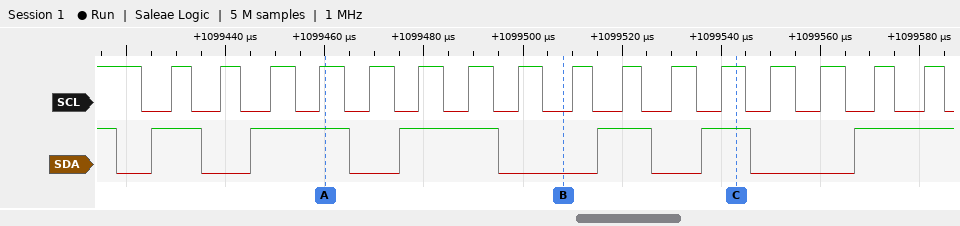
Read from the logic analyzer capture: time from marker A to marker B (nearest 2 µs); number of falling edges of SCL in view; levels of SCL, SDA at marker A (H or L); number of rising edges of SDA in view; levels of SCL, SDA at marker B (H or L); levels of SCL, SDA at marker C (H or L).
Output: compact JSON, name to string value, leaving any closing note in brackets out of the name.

{"time from marker A to marker B": "48 µs", "number of falling edges of SCL in view": "17", "levels of SCL, SDA at marker A": "SCL=H, SDA=H", "number of rising edges of SDA in view": "6", "levels of SCL, SDA at marker B": "SCL=L, SDA=L", "levels of SCL, SDA at marker C": "SCL=H, SDA=H"}
